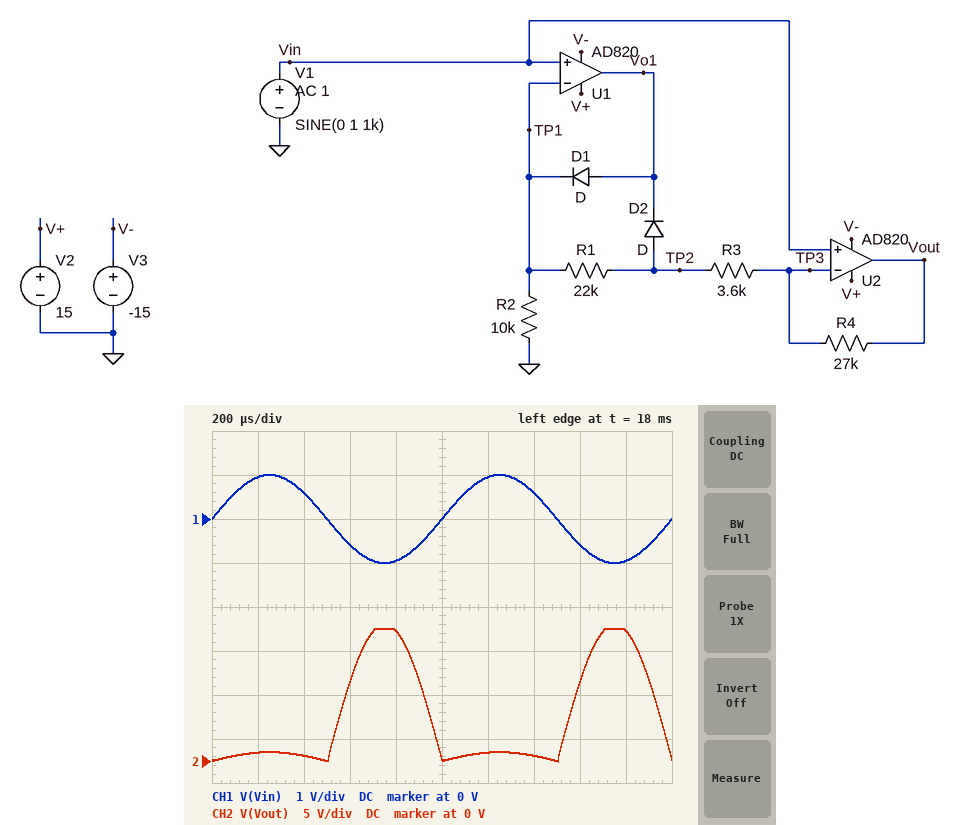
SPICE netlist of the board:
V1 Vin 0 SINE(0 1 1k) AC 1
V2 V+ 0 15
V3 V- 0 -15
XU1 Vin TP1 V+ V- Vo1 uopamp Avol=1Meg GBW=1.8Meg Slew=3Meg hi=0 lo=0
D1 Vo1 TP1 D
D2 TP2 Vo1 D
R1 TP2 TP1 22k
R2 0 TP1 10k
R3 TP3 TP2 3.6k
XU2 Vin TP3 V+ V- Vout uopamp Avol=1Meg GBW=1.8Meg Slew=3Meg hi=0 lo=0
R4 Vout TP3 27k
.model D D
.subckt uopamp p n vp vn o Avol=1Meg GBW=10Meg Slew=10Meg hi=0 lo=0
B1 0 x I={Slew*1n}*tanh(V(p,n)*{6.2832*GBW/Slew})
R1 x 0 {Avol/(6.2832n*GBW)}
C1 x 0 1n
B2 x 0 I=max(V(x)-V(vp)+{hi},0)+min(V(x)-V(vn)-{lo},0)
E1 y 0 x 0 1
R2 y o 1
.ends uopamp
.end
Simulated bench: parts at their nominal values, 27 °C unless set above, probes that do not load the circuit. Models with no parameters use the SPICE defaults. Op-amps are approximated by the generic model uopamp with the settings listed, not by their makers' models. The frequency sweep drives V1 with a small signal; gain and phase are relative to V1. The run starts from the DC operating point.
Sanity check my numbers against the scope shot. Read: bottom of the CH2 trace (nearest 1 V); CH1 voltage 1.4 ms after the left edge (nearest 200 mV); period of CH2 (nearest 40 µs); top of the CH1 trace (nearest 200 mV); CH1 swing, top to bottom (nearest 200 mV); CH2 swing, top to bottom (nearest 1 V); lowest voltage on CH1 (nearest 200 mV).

0 V
600 mV
1.00 ms
1.0 V
2.0 V
15 V
-1.0 V
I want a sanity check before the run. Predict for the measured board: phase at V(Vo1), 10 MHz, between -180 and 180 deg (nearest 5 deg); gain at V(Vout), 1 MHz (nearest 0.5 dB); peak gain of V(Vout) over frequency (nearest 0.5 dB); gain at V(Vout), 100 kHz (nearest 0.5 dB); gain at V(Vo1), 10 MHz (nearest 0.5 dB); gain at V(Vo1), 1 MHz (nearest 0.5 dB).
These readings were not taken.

-90 deg
2.0 dB
5.0 dB
5.0 dB
-15.0 dB
4.0 dB
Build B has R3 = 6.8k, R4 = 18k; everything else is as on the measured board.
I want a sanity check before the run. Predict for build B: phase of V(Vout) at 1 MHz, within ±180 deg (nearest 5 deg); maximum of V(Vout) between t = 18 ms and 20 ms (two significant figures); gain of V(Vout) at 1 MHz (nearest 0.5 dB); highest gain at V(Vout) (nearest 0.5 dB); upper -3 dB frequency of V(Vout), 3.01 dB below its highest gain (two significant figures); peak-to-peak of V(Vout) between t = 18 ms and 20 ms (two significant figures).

-40 deg
4.8 V
1.0 dB
3.5 dB
1.2 MHz
4.9 V
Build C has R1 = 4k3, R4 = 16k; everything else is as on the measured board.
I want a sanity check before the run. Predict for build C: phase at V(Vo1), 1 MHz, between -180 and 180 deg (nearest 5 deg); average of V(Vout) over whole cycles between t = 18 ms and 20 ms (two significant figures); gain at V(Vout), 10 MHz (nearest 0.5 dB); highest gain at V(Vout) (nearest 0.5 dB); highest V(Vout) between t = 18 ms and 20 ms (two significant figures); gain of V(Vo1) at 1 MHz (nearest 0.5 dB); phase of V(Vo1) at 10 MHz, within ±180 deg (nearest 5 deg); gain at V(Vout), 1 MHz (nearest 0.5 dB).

-70 deg
610 mV
-15.0 dB
5.5 dB
1.0 V
3.0 dB
-85 deg
2.5 dB
